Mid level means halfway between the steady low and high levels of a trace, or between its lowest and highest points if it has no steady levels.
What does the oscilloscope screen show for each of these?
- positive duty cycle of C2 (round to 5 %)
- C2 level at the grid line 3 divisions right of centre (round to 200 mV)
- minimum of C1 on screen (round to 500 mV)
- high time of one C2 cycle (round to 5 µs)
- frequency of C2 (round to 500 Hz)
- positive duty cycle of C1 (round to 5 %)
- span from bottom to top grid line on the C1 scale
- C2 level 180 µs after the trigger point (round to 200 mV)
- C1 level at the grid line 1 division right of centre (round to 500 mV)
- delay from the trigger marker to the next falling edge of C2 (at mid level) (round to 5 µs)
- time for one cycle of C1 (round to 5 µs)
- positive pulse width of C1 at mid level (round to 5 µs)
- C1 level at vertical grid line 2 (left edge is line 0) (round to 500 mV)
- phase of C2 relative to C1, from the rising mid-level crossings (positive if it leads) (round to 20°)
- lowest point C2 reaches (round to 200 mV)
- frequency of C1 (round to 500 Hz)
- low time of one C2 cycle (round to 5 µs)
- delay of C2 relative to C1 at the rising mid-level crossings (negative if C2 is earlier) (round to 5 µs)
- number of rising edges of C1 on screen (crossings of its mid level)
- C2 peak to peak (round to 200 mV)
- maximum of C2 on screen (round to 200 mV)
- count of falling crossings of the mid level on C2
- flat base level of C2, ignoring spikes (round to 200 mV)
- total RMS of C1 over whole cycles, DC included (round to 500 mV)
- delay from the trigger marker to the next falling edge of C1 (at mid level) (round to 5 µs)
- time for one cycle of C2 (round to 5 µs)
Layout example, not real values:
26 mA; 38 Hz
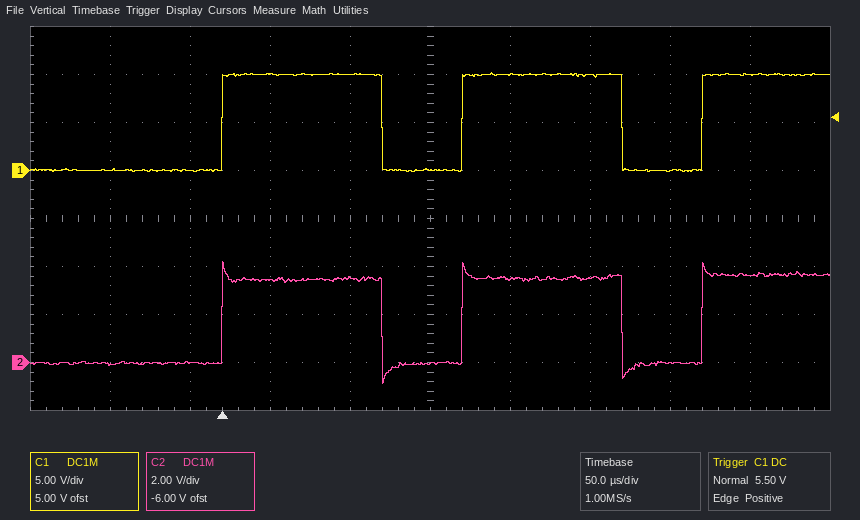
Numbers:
65 %; 0.0 V; 0.0 V; 100 µs; 6.5 kHz; 65 %; 40 V; 3.4 V; 10.0 V; 100 µs; 150 µs; 100 µs; 0.0 V; 0°; -800 mV; 6.5 kHz; 50 µs; 0 µs; 3; 5.0 V; 4.2 V; 2; 0.0 V; 8.0 V; 100 µs; 150 µs
